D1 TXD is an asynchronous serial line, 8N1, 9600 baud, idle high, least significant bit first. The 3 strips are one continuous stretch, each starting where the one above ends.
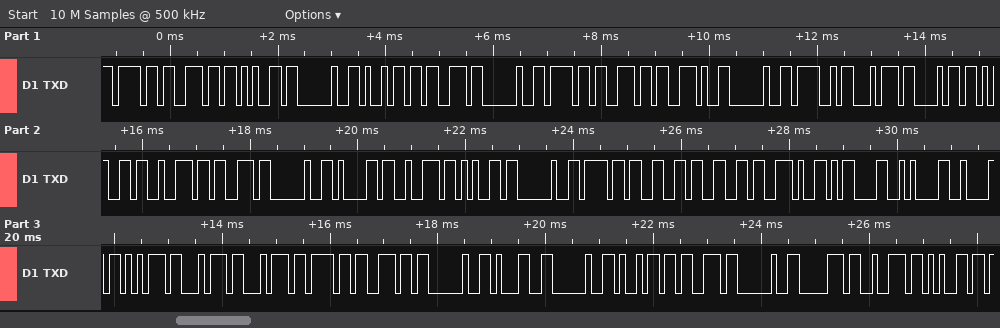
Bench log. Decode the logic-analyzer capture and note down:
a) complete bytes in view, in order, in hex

6F 6E 65 20 69 73 20 6F 6E 2E 20 4F 74 68 65 72 73 20 61 72 65 20 6F 66 66 2E 0D 0A 42 75 74 74 6F 6E 20 31 20 69 73 20 70 72 65
